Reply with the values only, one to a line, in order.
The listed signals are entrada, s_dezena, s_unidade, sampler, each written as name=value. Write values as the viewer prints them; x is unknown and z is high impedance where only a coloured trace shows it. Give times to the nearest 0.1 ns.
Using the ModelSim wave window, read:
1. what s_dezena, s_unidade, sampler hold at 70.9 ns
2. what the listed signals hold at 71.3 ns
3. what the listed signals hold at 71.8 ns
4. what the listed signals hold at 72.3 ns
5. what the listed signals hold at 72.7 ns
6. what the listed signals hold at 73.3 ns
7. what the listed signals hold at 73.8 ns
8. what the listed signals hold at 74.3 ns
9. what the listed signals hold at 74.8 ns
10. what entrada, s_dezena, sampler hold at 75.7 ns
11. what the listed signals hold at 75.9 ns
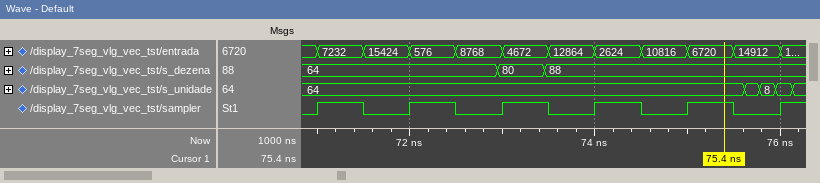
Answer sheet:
s_dezena=64, s_unidade=64, sampler=0
entrada=7232, s_dezena=64, s_unidade=64, sampler=1
entrada=15424, s_dezena=64, s_unidade=64, sampler=0
entrada=576, s_dezena=64, s_unidade=64, sampler=1
entrada=8768, s_dezena=64, s_unidade=64, sampler=0
entrada=4672, s_dezena=80, s_unidade=64, sampler=1
entrada=12864, s_dezena=88, s_unidade=64, sampler=0
entrada=2624, s_dezena=88, s_unidade=64, sampler=1
entrada=10816, s_dezena=88, s_unidade=64, sampler=0
entrada=14912, s_dezena=88, sampler=0
entrada=14912, s_dezena=88, s_unidade=8, sampler=0
